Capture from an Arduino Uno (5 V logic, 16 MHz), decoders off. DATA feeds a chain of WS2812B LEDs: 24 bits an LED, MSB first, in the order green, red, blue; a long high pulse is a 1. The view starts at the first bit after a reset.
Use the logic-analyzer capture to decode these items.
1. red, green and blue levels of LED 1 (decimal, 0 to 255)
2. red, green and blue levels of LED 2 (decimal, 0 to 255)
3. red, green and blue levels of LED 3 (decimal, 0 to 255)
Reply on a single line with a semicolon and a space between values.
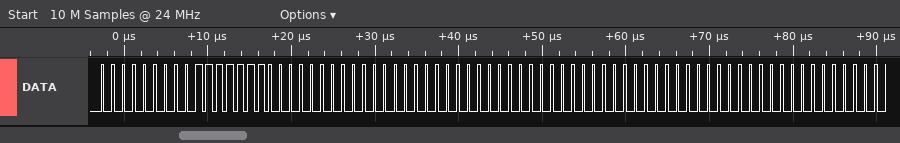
127, 0, 0; 0, 0, 0; 0, 0, 0
